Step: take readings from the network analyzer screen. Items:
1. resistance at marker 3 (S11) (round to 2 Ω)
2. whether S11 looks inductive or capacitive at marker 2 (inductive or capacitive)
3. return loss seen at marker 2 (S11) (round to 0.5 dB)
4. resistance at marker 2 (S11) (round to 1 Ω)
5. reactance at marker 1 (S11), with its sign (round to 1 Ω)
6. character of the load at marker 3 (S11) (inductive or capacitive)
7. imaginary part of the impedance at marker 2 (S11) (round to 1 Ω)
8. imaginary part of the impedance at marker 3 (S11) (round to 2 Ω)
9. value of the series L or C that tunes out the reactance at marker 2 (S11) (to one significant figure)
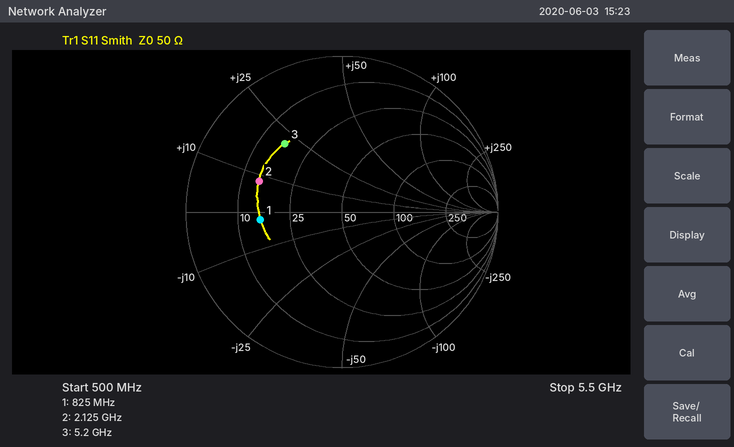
16 Ω
inductive
5.0 dB
14 Ω
-2 Ω
inductive
+8 Ω
+22 Ω
9 pF
